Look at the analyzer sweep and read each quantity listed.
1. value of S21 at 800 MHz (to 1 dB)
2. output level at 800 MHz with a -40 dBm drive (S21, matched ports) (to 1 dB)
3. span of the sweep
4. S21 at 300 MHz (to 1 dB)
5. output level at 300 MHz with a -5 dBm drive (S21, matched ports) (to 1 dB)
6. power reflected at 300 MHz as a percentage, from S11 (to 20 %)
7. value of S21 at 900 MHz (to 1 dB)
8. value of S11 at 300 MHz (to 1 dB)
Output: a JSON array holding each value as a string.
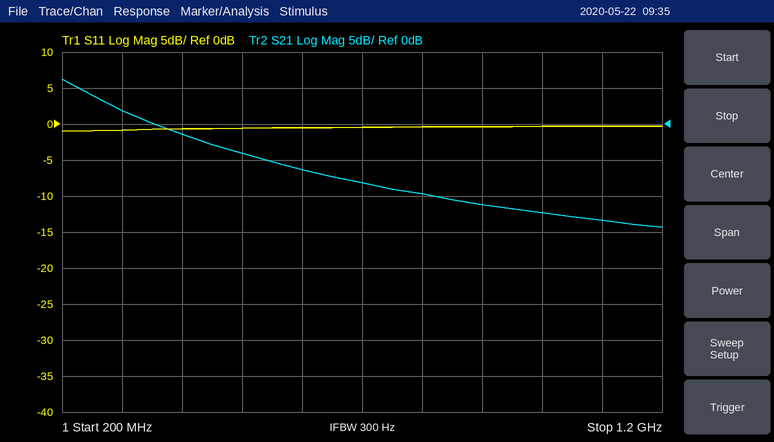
["-10 dB", "-50 dBm", "1 GHz", "2 dB", "-3 dBm", "80 %", "-11 dB", "-1 dB"]
